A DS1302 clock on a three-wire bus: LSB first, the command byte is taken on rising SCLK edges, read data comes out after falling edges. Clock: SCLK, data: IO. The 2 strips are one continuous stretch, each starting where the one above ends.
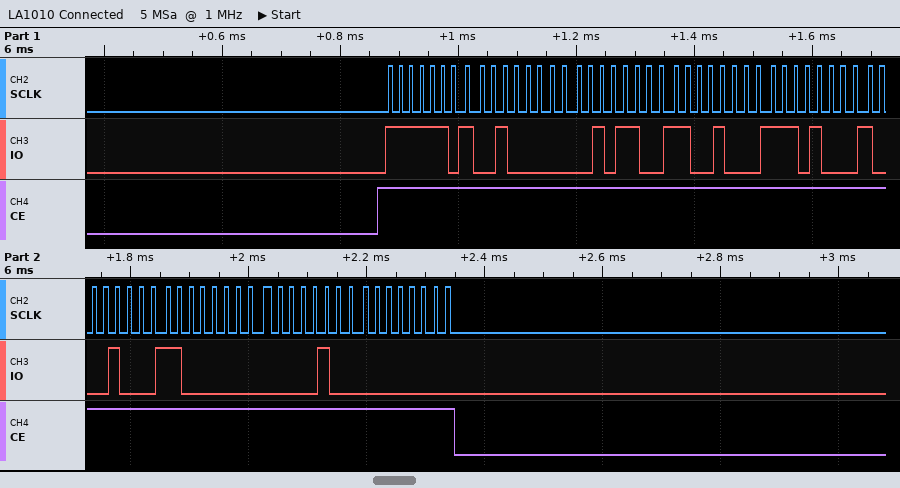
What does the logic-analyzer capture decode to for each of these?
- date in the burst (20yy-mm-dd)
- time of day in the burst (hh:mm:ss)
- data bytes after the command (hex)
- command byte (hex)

2020-11-17
13:34:04
04 34 13 17 11 03 20 00
0xBF
